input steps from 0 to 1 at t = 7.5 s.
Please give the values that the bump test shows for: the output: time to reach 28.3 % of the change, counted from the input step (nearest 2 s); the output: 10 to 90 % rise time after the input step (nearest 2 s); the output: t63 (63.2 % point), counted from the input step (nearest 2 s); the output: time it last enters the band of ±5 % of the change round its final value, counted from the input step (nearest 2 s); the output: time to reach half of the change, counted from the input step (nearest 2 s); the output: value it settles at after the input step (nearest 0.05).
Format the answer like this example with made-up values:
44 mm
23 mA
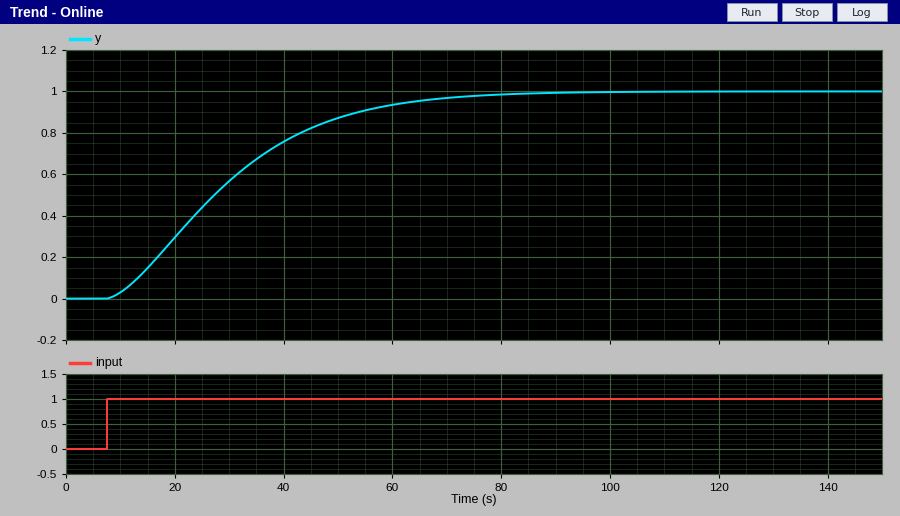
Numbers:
12 s
40 s
26 s
56 s
20 s
1.00
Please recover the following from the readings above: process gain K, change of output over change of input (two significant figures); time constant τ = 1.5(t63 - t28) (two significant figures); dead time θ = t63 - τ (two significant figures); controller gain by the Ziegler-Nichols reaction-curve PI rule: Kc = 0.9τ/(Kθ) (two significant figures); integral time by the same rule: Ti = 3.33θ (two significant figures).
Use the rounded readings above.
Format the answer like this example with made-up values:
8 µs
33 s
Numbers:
1.0
21 s
5.0 s
3.8
17 s
